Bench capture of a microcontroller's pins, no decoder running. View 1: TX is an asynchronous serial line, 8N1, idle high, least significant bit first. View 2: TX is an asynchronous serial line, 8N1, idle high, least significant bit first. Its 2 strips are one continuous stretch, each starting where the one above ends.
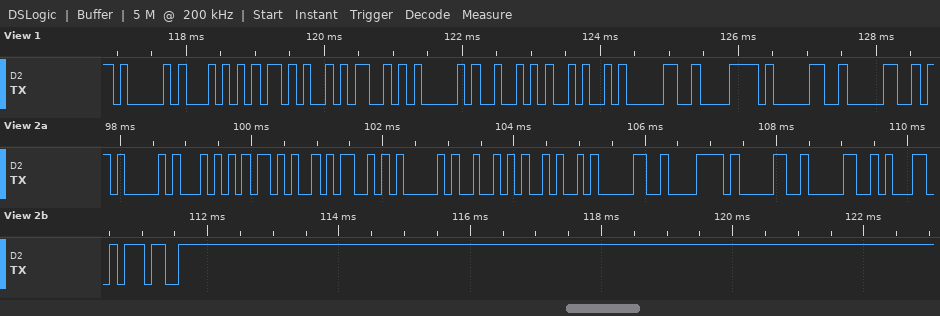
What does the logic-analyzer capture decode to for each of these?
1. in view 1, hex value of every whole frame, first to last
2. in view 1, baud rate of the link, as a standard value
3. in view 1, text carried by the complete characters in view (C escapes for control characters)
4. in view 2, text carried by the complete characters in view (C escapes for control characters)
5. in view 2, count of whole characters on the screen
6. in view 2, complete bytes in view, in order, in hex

41 54 2B 4D 41 52 4A 30 78 30 30
9600 baud
"AT+MARJ0x00"
"AT+MARJ0x0017"
13
41 54 2B 4D 41 52 4A 30 78 30 30 31 37
